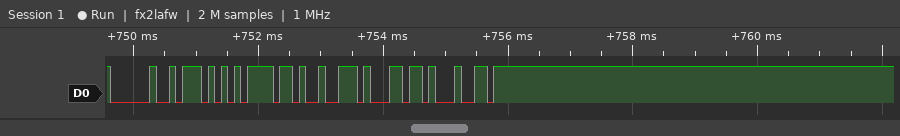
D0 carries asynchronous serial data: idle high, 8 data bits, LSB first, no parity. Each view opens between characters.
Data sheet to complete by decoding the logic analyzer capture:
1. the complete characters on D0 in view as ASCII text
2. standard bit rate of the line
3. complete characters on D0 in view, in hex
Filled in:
" World"
9600 baud
20, 57, 6F, 72, 6C, 64
